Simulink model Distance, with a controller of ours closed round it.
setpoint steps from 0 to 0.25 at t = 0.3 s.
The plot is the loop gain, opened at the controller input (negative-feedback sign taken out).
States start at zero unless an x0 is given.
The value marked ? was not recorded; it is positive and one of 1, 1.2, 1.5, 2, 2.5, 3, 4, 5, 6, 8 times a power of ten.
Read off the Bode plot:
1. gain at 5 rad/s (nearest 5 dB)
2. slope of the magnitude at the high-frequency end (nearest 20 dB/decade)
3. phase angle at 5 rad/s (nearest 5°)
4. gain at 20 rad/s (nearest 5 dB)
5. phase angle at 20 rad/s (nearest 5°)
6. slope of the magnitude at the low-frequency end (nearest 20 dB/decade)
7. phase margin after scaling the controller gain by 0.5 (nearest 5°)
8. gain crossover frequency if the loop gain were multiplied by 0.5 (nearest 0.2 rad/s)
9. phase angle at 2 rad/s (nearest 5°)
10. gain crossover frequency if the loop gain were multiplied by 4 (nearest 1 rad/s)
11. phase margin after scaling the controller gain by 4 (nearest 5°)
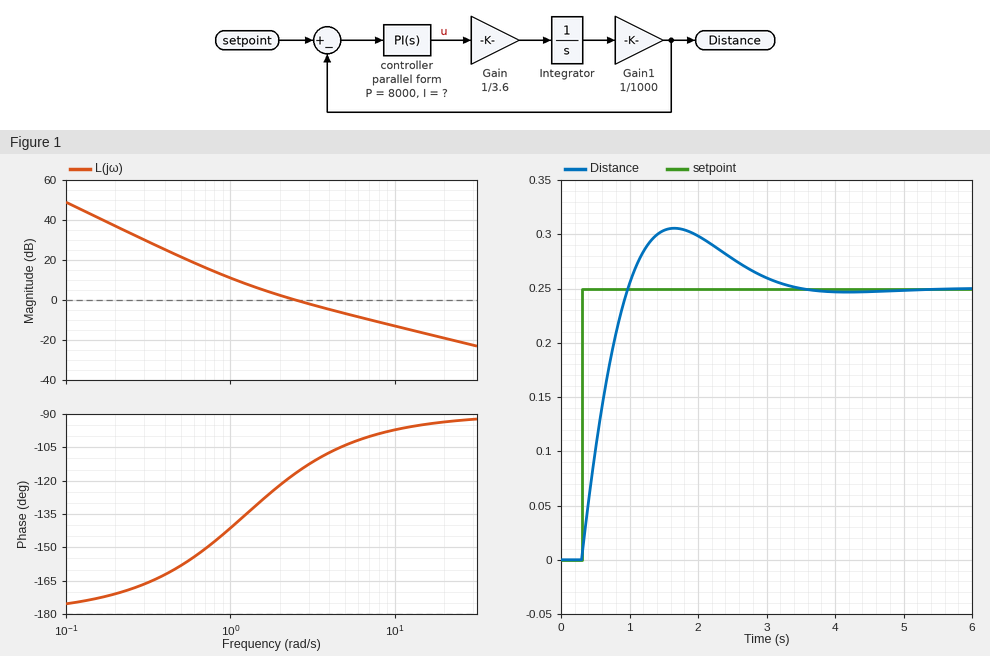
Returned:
-5 dB
-20 dB/decade
-105°
-20 dB
-95°
-40 dB/decade
50°
1.4 rad/s
-120°
9 rad/s
80°
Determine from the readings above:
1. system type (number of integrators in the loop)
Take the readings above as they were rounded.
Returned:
2
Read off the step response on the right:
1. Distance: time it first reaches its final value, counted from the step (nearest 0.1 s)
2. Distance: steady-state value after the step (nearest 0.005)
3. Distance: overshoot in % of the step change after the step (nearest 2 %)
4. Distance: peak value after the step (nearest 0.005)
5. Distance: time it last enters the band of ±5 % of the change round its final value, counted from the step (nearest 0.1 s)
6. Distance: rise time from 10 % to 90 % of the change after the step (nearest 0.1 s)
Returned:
0.7 s
0.250
22 %
0.305
2.6 s
0.5 s
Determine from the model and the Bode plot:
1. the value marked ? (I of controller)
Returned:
10000
